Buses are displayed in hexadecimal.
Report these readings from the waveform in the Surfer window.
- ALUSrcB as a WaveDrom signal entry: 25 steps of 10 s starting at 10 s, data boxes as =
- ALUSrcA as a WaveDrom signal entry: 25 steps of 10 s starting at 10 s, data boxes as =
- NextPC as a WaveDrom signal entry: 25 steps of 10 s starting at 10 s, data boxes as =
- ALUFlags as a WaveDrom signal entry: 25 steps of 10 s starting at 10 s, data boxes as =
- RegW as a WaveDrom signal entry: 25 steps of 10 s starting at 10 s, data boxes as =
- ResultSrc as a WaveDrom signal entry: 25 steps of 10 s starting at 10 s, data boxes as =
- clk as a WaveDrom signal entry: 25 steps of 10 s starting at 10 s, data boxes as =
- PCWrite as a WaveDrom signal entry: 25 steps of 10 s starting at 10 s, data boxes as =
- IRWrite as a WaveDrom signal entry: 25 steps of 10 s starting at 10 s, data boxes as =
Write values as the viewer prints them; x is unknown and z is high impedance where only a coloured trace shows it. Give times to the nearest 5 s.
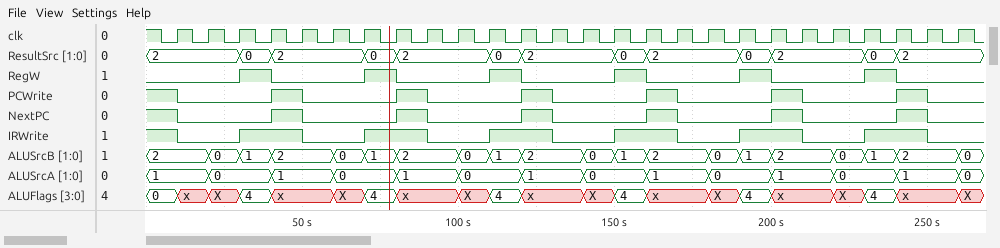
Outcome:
{name: 'ALUSrcB', wave: '====.===.===.===.===.===.', data: '2 0 1 2 0 1 2 0 1 2 0 1 2 0 1 2 0 1 2'}
{name: 'ALUSrcA', wave: '==.=.=.=.=.=.=.=.=.=.=.=.', data: '1 0 1 0 1 0 1 0 1 0 1 0 1'}
{name: 'NextPC', wave: '0..10..10..10..10..10..10'}
{name: 'ALUFlags', wave: 'x==x.==x.==x.==x.==x.==x.', data: 'X 4 X 4 X 4 X 4 X 4 X 4'}
{name: 'RegW', wave: '0.10..10..10..10..10..10.'}
{name: 'ResultSrc', wave: '=.==..==..==..==..==..==.', data: '2 0 2 0 2 0 2 0 2 0 2 0 2'}
{name: 'clk', wave: 'p........................'}
{name: 'PCWrite', wave: '0..10..10..10..10..10..10'}
{name: 'IRWrite', wave: '0.1.0.1.0.1.0.1.0.1.0.1.0'}
